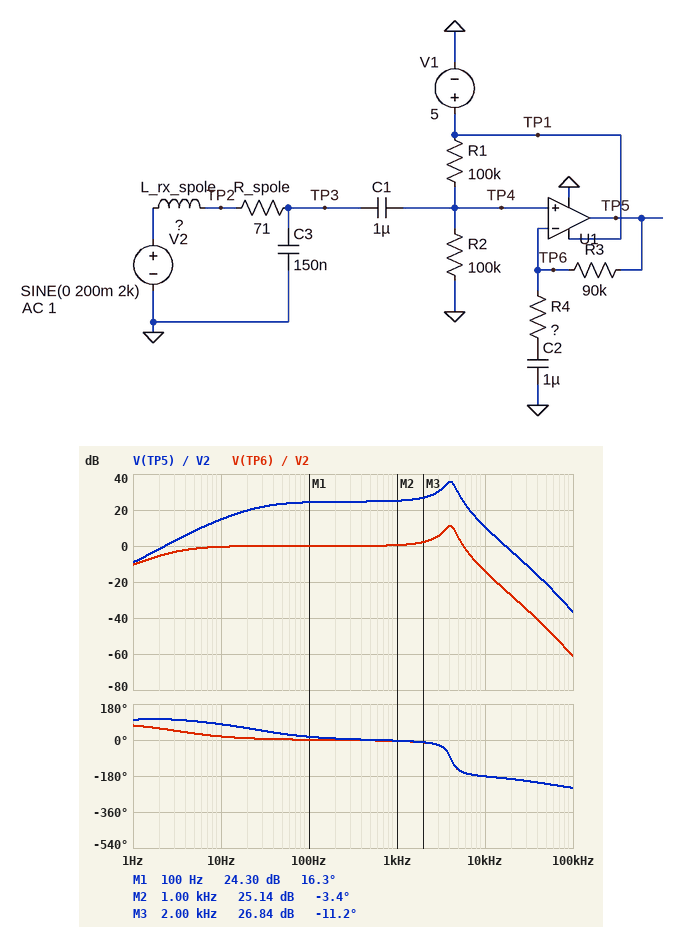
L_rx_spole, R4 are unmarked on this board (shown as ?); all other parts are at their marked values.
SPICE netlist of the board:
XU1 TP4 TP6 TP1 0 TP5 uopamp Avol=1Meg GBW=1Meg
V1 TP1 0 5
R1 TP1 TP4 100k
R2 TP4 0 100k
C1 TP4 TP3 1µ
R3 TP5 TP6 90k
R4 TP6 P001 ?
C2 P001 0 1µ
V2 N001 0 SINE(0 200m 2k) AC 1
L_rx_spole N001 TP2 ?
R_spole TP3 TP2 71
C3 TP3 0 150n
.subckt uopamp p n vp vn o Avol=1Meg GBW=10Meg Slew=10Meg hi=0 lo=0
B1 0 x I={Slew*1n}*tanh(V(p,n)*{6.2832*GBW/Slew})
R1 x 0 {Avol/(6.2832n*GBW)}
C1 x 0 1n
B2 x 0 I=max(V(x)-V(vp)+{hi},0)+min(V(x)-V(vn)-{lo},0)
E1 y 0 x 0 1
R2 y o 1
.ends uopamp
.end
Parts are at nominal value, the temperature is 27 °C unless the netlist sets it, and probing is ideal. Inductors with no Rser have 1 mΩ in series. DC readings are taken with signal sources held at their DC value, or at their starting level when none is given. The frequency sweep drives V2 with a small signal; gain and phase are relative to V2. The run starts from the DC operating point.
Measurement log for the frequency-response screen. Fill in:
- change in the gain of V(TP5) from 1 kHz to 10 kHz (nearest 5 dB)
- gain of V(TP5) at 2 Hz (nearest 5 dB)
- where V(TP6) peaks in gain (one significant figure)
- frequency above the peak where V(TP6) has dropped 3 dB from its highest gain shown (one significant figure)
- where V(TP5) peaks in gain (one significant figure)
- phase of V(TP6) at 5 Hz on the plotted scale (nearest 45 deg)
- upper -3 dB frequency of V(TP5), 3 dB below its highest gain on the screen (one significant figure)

-15 dB
0 dB
4 kHz
5 kHz
4 kHz
45 deg
5 kHz
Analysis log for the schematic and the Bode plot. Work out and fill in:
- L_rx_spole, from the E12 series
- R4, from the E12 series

10 mH
5.6 kΩ
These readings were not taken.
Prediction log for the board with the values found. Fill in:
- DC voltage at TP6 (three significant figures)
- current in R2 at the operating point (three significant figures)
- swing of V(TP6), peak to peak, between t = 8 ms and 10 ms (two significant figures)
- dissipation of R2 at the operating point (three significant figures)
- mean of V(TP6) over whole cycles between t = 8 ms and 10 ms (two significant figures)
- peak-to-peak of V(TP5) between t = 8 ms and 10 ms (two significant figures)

2.50 V
25.0 µA
300 mV
62.5 µW
2.5 V
5.0 V
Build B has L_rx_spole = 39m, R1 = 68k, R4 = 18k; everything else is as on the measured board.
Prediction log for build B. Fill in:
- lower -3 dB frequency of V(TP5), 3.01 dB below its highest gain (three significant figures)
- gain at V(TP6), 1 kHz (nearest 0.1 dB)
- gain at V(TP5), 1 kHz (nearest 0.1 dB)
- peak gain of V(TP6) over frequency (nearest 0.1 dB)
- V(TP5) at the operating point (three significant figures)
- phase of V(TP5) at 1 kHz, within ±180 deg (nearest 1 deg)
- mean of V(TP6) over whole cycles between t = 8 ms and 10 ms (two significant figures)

1.91 kHz
2.2 dB
17.8 dB
16.4 dB
2.98 V
-5 deg
2.9 V
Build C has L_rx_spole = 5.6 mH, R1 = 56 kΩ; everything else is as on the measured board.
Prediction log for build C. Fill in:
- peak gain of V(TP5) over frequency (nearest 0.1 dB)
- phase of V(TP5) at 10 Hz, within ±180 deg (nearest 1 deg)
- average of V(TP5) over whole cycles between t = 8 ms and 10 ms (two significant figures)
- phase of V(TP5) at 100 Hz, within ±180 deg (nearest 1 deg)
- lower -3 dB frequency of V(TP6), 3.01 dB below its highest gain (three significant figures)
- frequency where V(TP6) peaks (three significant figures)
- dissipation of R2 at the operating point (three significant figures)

33.3 dB
85 deg
3.0 V
17 deg
4.13 kHz
5.30 kHz
103 µW
